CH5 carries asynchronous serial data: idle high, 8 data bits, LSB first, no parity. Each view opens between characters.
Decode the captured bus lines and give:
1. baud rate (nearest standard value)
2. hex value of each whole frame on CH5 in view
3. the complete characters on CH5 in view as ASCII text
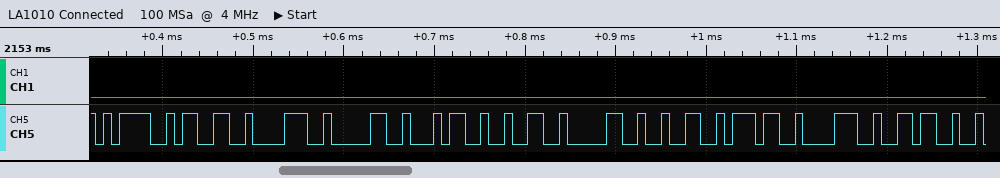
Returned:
115200 baud
3D, 33, 38, 30, 34, 32, 30, 32, 37, 38, 36
"=3804202786"
